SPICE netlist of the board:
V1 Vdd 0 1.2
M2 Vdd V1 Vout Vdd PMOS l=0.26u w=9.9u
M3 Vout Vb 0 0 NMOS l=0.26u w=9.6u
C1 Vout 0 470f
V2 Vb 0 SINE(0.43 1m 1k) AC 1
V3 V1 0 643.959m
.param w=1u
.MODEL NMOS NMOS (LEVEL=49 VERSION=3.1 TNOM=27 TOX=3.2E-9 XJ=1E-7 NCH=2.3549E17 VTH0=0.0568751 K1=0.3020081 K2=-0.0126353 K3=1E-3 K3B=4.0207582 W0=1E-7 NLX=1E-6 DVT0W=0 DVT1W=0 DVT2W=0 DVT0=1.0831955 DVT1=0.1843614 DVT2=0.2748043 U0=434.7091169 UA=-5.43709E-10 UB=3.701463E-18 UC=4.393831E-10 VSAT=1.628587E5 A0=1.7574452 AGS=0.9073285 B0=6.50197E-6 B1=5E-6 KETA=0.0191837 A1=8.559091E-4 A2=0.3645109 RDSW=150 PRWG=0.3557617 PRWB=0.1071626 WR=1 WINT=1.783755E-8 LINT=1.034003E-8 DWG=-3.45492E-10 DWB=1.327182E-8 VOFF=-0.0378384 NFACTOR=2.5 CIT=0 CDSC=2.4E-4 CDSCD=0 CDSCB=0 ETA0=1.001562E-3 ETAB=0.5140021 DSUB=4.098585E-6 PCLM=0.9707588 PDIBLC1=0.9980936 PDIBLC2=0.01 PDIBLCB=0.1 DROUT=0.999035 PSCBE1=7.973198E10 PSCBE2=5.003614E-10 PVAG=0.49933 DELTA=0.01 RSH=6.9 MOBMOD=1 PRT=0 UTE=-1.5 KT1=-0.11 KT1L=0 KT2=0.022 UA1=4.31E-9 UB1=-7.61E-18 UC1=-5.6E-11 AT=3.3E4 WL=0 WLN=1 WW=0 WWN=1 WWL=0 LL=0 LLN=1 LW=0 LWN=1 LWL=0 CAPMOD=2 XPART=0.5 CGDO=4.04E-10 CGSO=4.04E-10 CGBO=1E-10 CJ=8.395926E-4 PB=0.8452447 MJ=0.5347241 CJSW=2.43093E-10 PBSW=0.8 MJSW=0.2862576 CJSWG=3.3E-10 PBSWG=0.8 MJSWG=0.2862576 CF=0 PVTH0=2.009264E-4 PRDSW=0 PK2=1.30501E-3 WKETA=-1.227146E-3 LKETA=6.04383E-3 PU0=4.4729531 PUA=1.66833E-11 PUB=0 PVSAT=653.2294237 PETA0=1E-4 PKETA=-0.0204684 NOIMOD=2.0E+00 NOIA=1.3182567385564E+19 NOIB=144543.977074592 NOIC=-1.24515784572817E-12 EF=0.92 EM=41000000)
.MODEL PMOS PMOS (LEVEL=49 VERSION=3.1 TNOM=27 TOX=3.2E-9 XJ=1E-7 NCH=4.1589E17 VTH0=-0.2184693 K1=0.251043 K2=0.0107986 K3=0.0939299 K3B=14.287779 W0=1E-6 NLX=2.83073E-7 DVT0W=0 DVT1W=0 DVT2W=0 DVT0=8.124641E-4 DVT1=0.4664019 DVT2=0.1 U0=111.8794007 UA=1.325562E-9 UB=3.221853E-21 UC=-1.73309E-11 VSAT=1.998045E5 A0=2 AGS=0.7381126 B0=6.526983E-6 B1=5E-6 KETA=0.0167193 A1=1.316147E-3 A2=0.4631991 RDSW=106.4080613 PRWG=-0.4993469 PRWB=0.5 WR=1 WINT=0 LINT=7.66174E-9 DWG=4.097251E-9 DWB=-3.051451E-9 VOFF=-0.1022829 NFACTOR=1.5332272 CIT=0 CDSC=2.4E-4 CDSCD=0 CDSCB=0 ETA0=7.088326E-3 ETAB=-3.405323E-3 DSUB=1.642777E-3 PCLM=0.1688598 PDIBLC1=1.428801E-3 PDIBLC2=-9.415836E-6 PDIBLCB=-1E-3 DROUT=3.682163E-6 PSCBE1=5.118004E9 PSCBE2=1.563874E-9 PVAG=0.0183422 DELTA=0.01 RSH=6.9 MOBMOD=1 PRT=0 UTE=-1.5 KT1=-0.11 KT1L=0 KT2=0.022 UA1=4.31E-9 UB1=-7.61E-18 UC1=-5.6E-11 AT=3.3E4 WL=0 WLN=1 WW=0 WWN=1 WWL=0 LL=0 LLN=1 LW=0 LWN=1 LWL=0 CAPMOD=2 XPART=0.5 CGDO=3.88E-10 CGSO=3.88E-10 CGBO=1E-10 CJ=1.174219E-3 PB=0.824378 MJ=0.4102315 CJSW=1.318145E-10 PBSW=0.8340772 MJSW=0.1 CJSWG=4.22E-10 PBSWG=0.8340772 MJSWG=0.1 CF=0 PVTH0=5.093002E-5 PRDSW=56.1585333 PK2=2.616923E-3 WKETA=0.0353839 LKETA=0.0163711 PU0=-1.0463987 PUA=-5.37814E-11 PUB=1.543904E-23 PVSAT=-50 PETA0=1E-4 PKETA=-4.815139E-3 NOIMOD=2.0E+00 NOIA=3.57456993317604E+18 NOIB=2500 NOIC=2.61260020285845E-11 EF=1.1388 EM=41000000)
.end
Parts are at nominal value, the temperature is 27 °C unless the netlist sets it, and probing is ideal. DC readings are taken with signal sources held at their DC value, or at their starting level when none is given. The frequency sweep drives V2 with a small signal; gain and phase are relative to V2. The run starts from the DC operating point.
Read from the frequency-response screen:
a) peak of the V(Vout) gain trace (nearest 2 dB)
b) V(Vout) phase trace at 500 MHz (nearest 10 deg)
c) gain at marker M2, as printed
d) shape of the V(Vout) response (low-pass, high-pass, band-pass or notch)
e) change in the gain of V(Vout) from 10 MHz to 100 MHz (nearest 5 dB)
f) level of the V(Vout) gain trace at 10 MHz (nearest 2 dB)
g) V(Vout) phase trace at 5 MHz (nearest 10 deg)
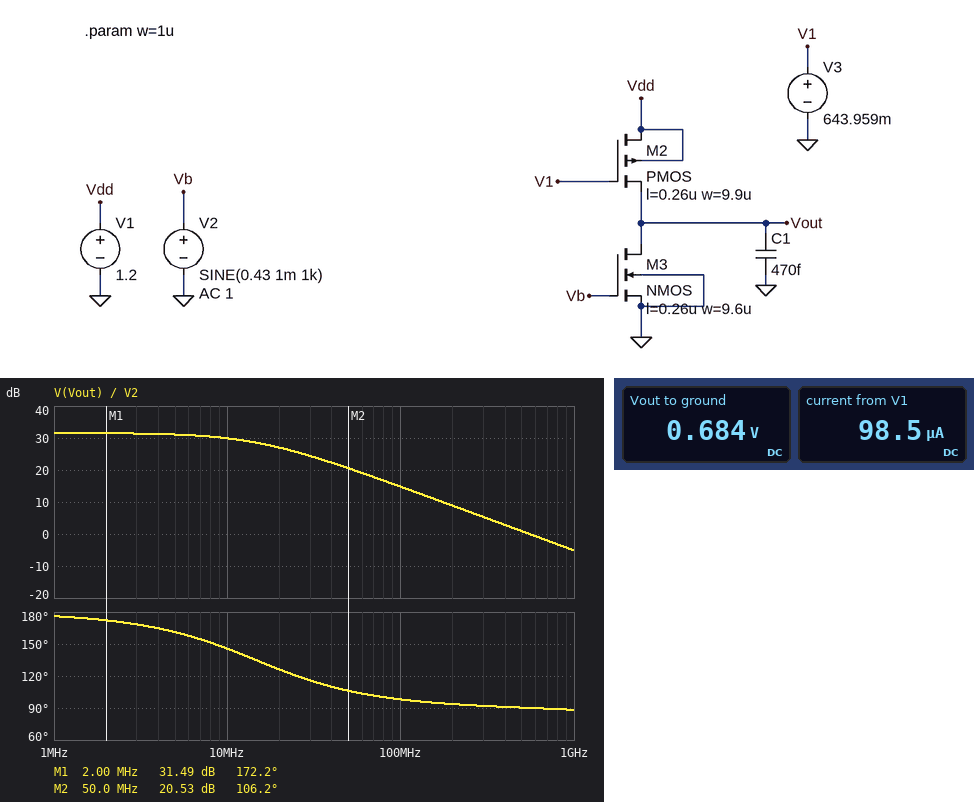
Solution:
32 dB
90 deg
20.53 dB
low-pass
-15 dB
30 dB
160 deg
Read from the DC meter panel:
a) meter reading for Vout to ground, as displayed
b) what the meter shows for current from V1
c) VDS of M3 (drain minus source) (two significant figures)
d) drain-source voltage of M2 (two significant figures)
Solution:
0.684 V
98.5 µA
680 mV
520 mV
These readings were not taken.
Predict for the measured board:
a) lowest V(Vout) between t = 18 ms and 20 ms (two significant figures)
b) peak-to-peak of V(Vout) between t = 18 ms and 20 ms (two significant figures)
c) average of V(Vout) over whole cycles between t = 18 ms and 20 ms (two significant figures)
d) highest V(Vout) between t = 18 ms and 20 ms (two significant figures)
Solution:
650 mV
76 mV
680 mV
720 mV
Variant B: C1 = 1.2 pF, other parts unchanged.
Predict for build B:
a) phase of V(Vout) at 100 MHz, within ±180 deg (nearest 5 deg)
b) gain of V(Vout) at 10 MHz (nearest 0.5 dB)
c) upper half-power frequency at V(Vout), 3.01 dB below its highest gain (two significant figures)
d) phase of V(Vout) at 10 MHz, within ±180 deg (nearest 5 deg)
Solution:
95 deg
25.5 dB
5.8 MHz
120 deg
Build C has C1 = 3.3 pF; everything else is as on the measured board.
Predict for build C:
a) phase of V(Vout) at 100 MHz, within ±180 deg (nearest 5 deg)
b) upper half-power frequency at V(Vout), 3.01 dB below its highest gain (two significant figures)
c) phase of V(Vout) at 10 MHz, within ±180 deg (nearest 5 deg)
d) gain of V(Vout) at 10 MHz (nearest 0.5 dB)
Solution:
90 deg
2.1 MHz
100 deg
18.0 dB
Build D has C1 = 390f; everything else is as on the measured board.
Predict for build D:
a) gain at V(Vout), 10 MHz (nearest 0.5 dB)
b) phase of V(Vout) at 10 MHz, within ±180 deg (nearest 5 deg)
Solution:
30.5 dB
150 deg
